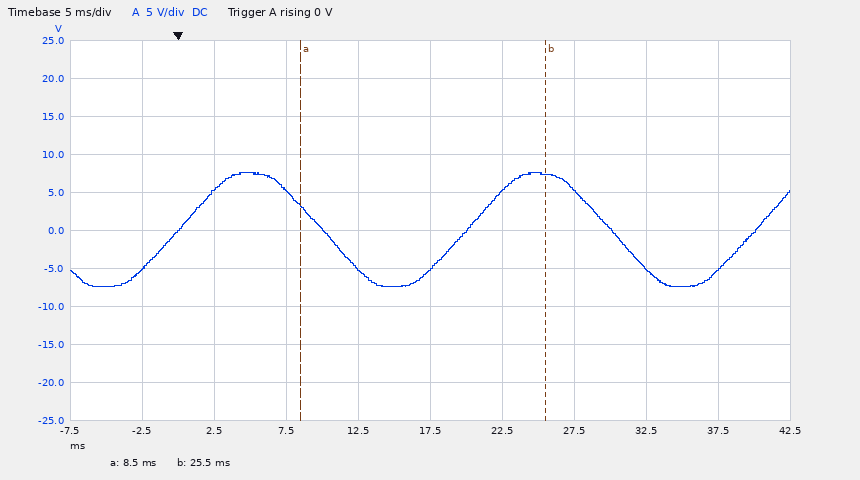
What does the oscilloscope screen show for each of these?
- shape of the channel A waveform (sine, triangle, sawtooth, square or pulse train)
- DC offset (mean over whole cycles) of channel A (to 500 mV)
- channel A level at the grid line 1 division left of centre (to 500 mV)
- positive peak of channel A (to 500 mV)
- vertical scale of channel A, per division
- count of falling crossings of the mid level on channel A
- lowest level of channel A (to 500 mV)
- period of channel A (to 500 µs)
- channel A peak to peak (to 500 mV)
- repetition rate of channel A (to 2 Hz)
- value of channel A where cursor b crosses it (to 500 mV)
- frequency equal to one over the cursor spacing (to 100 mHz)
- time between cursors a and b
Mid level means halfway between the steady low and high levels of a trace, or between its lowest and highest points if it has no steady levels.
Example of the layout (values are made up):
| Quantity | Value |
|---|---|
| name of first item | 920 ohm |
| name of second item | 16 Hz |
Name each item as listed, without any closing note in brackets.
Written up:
| Quantity | Value |
|---|---|
| shape of the channel A waveform | sine |
| DC offset (mean over whole cycles) of channel A | 0.0 V |
| channel A level at the grid line 1 division left of centre | -5.0 V |
| positive peak of channel A | 7.5 V |
| vertical scale of channel A, per division | 5 V |
| count of falling crossings of the mid level on channel A | 2 |
| lowest level of channel A | -7.5 V |
| period of channel A | 20.0 ms |
| channel A peak to peak | 15.0 V |
| repetition rate of channel A | 50 Hz |
| value of channel A where cursor b crosses it | 7.5 V |
| frequency equal to one over the cursor spacing | 58.8 Hz |
| time between cursors a and b | 17.0 ms |
